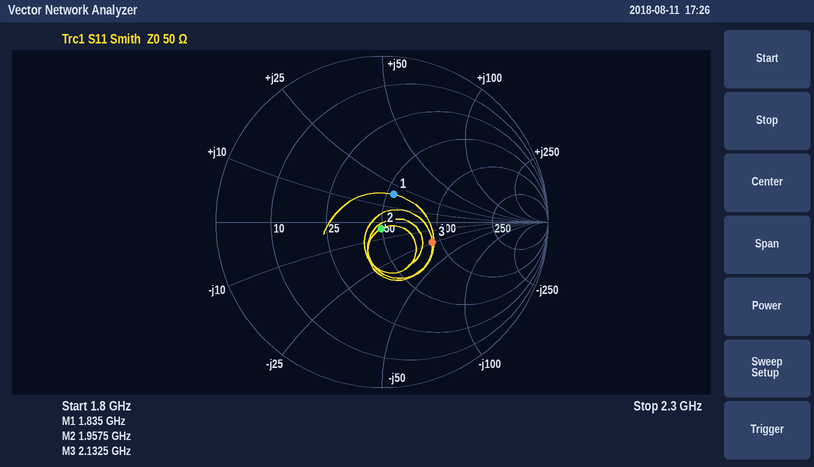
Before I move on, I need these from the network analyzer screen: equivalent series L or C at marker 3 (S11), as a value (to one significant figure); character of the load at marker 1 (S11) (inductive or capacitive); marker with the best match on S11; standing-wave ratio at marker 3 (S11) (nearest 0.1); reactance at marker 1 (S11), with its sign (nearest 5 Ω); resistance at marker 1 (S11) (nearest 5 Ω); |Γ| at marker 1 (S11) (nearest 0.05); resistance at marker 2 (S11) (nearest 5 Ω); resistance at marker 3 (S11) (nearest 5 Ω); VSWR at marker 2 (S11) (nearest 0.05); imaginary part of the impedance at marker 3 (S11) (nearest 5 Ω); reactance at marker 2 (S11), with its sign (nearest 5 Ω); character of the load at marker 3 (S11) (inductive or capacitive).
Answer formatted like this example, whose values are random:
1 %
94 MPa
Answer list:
3 pF
inductive
marker 2
2.0
+20 Ω
55 Ω
0.20
50 Ω
90 Ω
1.10
-25 Ω
-5 Ω
capacitive
